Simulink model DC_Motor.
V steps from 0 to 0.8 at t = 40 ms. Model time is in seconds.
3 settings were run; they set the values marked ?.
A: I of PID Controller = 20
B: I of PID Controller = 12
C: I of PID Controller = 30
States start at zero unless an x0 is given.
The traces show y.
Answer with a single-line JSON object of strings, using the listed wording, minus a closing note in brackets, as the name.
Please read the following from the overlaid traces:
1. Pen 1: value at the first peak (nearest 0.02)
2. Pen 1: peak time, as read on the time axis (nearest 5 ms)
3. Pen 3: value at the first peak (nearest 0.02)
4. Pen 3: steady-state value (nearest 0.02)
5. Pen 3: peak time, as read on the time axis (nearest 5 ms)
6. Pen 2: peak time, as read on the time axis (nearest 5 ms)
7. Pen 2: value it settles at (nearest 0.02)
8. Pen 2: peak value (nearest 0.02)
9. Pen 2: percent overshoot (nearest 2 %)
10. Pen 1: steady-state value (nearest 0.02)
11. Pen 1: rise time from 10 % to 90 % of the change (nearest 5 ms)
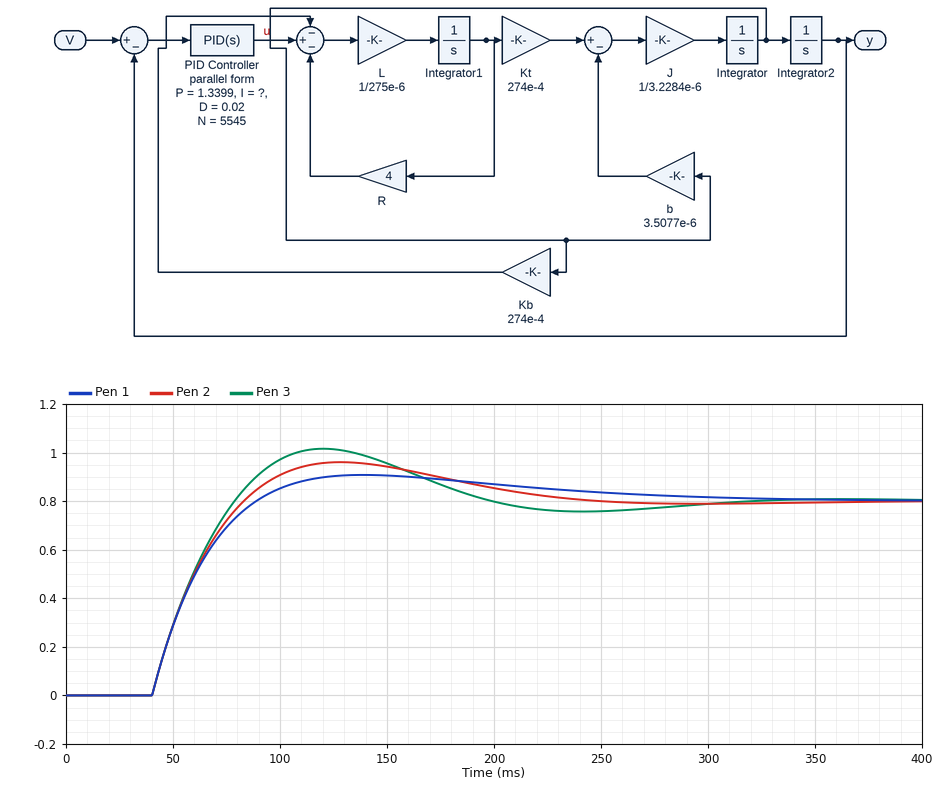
{"Pen 1: value at the first peak": "0.90", "Pen 1: peak time, as read on the time axis": "140 ms", "Pen 3: value at the first peak": "1.02", "Pen 3: steady-state value": "0.80", "Pen 3: peak time, as read on the time axis": "120 ms", "Pen 2: peak time, as read on the time axis": "130 ms", "Pen 2: value it settles at": "0.80", "Pen 2: peak value": "0.96", "Pen 2: percent overshoot": "20 %", "Pen 1: steady-state value": "0.80", "Pen 1: rise time from 10 % to 90 % of the change": "35 ms"}
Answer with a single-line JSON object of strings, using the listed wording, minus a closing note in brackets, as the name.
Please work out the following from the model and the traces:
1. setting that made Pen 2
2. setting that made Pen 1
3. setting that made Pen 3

{"setting that made Pen 2": "A", "setting that made Pen 1": "B", "setting that made Pen 3": "C"}
